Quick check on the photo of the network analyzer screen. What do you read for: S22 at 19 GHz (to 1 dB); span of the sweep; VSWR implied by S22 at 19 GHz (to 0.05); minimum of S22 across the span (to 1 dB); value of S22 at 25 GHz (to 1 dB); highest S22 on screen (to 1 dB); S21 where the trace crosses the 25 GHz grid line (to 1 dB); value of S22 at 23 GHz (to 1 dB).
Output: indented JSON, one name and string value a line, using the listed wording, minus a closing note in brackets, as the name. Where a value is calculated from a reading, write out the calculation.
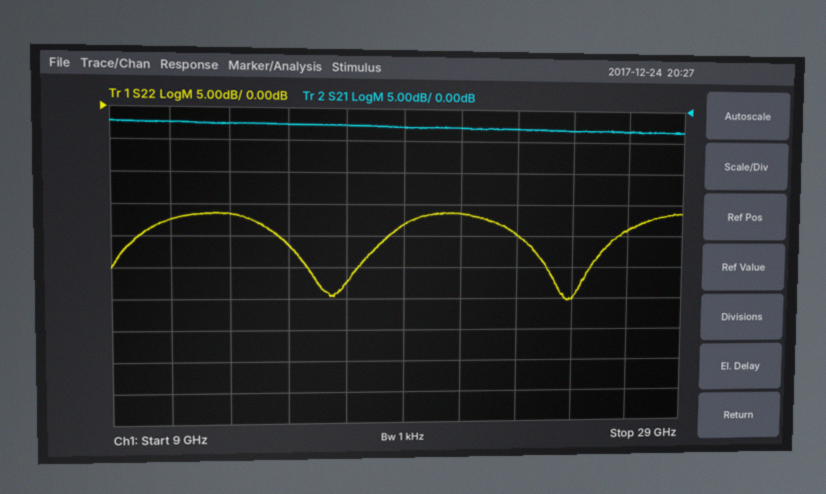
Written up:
{
  "S22 at 19 GHz": "-18 dB",
  "span of the sweep": "20 GHz",
  "VSWR implied by S22 at 19 GHz": "|Γ| = 10^(-18/20) = 0.1259; VSWR = (1 + 0.1259)/(1 − 0.1259) ≈ 1.29, so 1.30 to the nearest 0.05",
  "minimum of S22 across the span": "-30 dB",
  "value of S22 at 25 GHz": "-30 dB",
  "highest S22 on screen": "-16 dB",
  "S21 where the trace crosses the 25 GHz grid line": "-3 dB",
  "value of S22 at 23 GHz": "-20 dB"
}
